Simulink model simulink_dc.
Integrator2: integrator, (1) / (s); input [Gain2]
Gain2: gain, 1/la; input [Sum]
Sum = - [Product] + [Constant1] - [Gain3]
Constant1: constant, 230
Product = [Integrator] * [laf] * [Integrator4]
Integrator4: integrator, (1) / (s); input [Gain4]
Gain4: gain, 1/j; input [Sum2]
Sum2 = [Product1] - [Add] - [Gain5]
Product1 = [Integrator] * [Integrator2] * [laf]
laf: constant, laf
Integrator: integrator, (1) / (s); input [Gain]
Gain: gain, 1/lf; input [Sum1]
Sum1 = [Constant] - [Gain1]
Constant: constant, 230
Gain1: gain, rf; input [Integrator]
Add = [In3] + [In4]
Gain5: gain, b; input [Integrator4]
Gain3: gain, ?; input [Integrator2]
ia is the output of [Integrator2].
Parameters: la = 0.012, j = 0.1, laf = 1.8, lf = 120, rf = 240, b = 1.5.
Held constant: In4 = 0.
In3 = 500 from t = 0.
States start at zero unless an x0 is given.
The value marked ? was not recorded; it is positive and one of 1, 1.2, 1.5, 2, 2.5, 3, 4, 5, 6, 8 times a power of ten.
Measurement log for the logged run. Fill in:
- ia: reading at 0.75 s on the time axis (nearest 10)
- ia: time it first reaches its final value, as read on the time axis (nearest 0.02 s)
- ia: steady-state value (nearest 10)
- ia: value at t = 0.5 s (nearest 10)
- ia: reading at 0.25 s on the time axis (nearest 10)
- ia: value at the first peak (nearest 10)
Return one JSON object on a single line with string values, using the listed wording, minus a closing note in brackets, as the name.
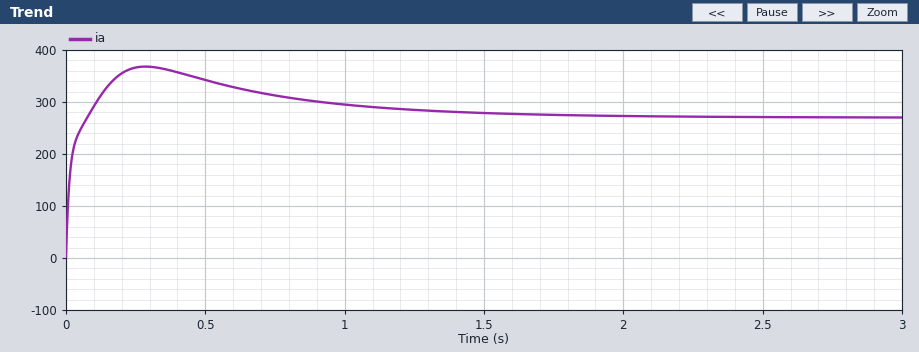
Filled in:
{"ia: reading at 0.75 s on the time axis": "310", "ia: time it first reaches its final value, as read on the time axis": "0.08 s", "ia: steady-state value": "270", "ia: value at t = 0.5 s": "340", "ia: reading at 0.25 s on the time axis": "370", "ia: value at the first peak": "370"}
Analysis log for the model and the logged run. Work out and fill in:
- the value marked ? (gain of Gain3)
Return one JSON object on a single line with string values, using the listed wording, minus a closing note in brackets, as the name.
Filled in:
{"the value marked ?": "1"}
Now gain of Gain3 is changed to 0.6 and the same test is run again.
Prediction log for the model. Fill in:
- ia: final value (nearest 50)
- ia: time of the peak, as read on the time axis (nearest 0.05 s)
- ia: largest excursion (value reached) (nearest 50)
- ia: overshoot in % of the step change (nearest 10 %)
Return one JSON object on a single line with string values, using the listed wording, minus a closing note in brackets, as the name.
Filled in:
{"ia: final value": "300", "ia: time of the peak, as read on the time axis": "0.20 s", "ia: largest excursion (value reached)": "550", "ia: overshoot in % of the step change": "80 %"}
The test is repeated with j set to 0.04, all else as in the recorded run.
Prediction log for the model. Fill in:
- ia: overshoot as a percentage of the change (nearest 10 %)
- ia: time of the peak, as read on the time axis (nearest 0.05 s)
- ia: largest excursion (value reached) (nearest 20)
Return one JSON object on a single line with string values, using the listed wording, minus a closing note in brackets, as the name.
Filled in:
{"ia: overshoot as a percentage of the change": "30 %", "ia: time of the peak, as read on the time axis": "0.25 s", "ia: largest excursion (value reached)": "360"}
